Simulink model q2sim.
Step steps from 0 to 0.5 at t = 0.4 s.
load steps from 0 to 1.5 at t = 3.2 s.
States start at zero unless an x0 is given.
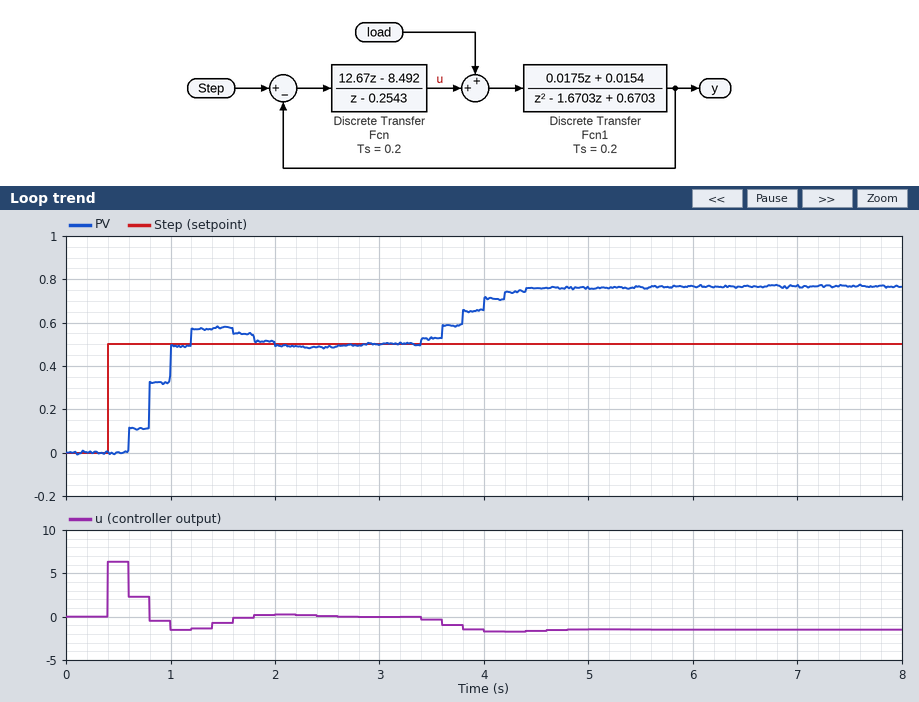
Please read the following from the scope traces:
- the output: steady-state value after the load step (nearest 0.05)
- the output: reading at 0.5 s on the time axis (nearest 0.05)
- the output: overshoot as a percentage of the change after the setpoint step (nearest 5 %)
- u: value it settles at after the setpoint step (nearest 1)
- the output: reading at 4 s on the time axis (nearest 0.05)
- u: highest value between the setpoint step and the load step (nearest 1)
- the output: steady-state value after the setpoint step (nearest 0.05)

0.75
0.00
15 %
0
0.70
6
0.50
